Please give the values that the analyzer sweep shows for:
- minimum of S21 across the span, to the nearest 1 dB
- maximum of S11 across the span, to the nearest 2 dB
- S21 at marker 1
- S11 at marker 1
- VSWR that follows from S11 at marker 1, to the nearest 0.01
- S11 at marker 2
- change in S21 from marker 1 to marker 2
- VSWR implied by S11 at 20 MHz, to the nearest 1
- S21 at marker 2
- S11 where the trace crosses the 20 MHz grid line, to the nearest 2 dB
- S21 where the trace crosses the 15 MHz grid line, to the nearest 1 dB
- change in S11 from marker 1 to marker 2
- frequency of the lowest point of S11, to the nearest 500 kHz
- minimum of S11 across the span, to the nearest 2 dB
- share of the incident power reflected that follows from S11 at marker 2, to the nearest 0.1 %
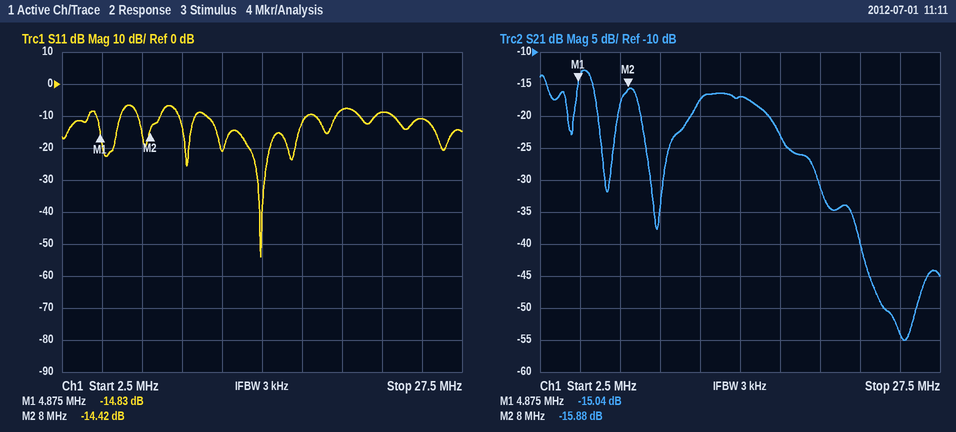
-55 dB
-6 dB
-15.04 dB
-14.83 dB
1.44
-14.42 dB
-0.84 dB
2
-15.88 dB
-8 dB
-17 dB
0.41 dB
15.0 MHz
-54 dB
3.6 %
